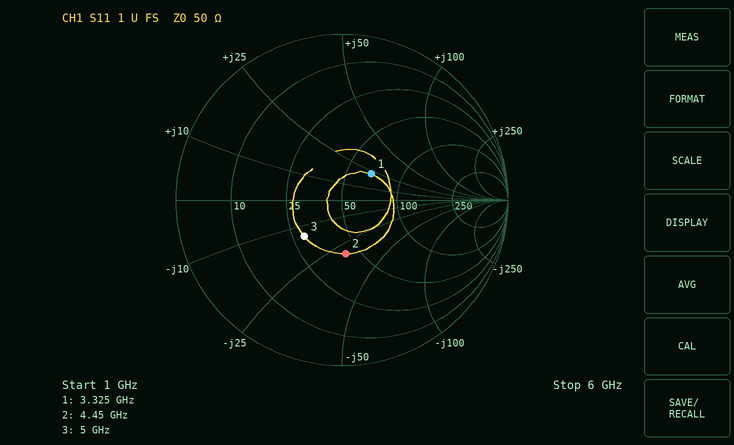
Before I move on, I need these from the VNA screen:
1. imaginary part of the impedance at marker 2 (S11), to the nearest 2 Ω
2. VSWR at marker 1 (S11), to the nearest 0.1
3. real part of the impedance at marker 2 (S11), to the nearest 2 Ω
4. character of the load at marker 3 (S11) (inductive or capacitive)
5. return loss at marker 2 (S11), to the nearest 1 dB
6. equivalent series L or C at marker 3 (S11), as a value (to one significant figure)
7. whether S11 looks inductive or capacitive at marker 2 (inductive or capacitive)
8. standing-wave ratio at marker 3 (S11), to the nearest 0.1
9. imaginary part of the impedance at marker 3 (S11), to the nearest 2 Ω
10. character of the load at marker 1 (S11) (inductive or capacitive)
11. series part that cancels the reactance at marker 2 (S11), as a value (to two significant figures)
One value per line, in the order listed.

-30 Ω
1.6
42 Ω
capacitive
10 dB
2 pF
capacitive
1.9
-14 Ω
inductive
1.1 nH
